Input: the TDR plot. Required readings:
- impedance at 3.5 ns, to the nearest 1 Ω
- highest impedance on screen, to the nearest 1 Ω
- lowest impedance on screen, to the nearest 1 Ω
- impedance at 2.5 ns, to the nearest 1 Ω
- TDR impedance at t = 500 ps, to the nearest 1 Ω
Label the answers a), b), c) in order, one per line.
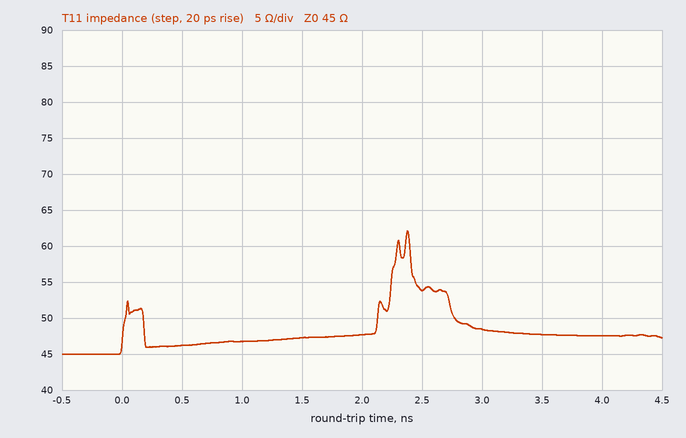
a) 48 Ω
b) 62 Ω
c) 45 Ω
d) 54 Ω
e) 46 Ω
